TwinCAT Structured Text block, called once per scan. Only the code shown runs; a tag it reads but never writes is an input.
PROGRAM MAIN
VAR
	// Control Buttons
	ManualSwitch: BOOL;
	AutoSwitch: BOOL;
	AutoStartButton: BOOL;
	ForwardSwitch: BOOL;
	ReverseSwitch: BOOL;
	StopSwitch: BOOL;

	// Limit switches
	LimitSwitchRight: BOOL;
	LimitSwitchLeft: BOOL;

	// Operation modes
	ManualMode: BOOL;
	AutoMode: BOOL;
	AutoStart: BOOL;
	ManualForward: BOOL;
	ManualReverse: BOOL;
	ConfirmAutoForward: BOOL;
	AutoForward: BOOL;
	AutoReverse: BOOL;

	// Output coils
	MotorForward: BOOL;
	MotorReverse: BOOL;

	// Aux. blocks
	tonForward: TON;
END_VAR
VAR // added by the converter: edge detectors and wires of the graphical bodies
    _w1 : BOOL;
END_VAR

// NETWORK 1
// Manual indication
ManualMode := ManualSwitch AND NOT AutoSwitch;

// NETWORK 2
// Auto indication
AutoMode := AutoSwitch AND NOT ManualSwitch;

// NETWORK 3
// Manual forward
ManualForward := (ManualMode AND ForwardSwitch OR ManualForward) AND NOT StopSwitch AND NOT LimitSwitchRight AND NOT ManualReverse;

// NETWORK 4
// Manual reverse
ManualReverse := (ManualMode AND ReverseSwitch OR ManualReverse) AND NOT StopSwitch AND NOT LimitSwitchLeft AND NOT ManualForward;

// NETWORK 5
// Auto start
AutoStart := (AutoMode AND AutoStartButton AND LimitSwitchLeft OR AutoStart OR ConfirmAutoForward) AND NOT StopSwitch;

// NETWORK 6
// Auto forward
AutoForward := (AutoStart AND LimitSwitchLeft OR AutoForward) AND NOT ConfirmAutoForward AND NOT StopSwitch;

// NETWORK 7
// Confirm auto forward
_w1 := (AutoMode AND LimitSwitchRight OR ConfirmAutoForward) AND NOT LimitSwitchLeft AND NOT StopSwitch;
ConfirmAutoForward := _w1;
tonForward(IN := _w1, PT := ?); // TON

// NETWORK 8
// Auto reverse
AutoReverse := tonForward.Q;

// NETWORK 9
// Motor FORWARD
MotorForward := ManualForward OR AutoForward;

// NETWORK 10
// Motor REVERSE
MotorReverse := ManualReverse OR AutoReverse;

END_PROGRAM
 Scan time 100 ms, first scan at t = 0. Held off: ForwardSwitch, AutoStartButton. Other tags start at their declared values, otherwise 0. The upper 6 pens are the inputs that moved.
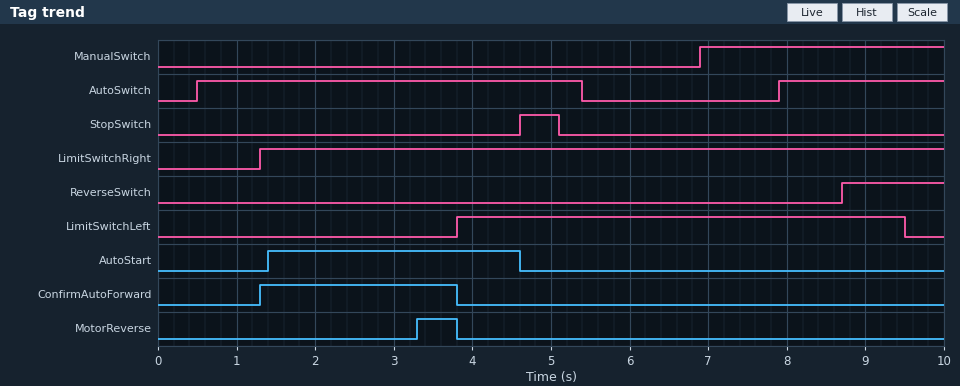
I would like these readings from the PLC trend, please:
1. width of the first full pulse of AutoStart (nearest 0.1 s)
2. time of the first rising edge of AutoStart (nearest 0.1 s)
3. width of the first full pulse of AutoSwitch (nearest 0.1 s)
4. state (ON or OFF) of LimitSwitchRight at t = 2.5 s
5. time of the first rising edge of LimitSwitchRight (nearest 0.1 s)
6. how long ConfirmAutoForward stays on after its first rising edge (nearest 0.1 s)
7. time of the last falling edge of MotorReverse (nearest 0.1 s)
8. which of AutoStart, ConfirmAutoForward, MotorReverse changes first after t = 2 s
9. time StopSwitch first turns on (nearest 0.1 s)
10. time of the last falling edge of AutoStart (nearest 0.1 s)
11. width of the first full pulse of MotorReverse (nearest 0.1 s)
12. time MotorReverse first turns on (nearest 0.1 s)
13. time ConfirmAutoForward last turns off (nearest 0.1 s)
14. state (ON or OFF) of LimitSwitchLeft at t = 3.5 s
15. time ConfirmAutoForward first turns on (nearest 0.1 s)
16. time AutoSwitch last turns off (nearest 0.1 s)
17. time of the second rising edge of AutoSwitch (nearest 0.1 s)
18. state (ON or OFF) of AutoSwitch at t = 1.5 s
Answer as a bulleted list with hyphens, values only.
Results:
- 3.2 s
- 1.4 s
- 4.9 s
- ON
- 1.3 s
- 2.5 s
- 3.8 s
- MotorReverse
- 4.6 s
- 4.6 s
- 0.5 s
- 3.3 s
- 3.8 s
- OFF
- 1.3 s
- 5.4 s
- 7.9 s
- ON
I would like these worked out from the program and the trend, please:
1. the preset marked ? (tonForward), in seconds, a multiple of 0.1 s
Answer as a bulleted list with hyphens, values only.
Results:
- 2.0 s
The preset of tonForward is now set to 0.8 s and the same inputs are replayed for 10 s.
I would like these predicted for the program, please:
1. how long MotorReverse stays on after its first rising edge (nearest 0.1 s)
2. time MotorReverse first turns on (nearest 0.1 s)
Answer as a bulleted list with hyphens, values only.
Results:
- 1.7 s
- 2.1 s
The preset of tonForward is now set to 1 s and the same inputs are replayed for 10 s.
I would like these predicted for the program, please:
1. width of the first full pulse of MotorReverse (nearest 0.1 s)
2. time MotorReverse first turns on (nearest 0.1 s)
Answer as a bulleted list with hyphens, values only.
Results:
- 1.5 s
- 2.3 s
